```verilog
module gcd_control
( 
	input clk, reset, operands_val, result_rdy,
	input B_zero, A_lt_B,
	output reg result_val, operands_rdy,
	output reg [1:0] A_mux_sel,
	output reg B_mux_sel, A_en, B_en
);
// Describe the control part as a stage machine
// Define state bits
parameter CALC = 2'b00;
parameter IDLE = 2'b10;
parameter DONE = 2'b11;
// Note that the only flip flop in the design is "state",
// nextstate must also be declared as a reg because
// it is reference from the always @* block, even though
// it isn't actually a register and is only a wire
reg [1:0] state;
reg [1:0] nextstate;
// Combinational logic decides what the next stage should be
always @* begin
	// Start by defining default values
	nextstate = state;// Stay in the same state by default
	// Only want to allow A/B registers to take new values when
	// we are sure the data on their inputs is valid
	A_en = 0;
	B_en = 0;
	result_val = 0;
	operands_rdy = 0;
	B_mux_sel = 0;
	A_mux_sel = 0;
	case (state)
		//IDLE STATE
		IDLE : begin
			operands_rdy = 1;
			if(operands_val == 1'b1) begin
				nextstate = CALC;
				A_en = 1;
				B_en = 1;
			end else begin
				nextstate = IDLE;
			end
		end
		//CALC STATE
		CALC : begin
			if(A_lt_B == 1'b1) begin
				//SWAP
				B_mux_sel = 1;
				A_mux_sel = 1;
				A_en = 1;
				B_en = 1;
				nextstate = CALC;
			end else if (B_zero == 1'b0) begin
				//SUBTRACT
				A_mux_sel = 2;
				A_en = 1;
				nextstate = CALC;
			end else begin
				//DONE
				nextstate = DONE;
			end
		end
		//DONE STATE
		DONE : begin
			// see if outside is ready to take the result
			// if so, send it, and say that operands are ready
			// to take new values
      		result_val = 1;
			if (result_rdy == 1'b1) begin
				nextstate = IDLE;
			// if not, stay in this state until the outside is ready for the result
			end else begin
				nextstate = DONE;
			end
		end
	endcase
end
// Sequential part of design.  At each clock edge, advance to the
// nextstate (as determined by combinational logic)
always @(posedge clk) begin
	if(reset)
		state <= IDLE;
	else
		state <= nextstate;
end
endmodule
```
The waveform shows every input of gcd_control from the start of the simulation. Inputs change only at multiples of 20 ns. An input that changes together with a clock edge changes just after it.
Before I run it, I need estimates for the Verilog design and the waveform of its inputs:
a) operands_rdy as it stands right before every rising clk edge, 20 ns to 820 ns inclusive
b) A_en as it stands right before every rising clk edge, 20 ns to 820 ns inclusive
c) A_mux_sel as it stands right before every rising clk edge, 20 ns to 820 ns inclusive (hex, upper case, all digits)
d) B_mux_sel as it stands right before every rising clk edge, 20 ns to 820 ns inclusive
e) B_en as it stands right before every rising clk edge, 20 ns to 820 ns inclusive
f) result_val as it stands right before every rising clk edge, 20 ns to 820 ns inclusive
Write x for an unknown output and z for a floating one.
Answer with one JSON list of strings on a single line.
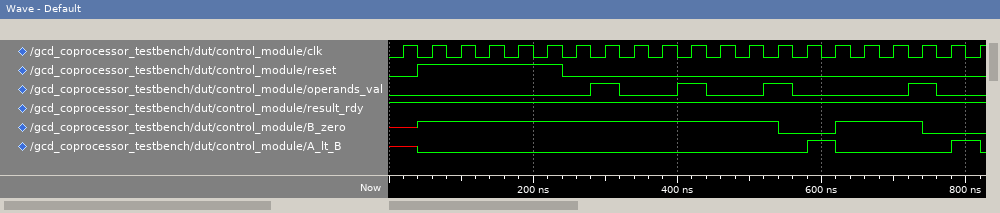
["0 0 1 1 1 1 1 1 0 0 1 0 0 1 0 0 0 0 1 0 0", "0 0 0 0 0 0 0 1 0 0 1 0 0 1 1 1 0 0 1 1 1", "0, 0, 0, 0, 0, 0, 0, 0, 0, 0, 0, 0, 0, 0, 2, 1, 0, 0, 0, 2, 1", "0 0 0 0 0 0 0 0 0 0 0 0 0 0 0 1 0 0 0 0 1", "0 0 0 0 0 0 0 1 0 0 1 0 0 1 0 1 0 0 1 0 1", "0 0 0 0 0 0 0 0 0 1 0 0 1 0 0 0 0 1 0 0 0"]
